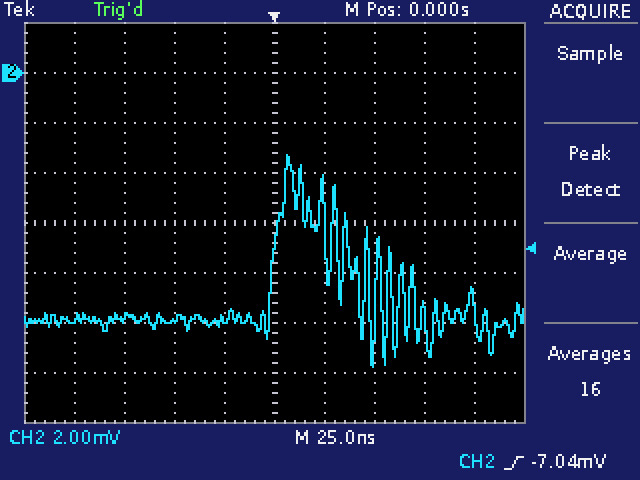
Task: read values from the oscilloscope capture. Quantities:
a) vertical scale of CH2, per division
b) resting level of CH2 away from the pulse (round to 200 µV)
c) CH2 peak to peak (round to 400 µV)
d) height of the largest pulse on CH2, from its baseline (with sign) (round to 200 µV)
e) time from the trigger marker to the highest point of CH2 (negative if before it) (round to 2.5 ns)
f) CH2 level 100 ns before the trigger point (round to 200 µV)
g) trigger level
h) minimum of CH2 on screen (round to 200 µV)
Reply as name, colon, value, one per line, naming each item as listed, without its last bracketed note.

vertical scale of CH2, per division: 2 mV
resting level of CH2 away from the pulse: -9.8 mV
CH2 peak to peak: 8.4 mV
height of the largest pulse on CH2, from its baseline (with sign): +6.6 mV
time from the trigger marker to the highest point of CH2 (negative if before it): +7.5 ns
CH2 level 100 ns before the trigger point: -9.8 mV
trigger level: -7.04 mV
minimum of CH2 on screen: -11.8 mV
